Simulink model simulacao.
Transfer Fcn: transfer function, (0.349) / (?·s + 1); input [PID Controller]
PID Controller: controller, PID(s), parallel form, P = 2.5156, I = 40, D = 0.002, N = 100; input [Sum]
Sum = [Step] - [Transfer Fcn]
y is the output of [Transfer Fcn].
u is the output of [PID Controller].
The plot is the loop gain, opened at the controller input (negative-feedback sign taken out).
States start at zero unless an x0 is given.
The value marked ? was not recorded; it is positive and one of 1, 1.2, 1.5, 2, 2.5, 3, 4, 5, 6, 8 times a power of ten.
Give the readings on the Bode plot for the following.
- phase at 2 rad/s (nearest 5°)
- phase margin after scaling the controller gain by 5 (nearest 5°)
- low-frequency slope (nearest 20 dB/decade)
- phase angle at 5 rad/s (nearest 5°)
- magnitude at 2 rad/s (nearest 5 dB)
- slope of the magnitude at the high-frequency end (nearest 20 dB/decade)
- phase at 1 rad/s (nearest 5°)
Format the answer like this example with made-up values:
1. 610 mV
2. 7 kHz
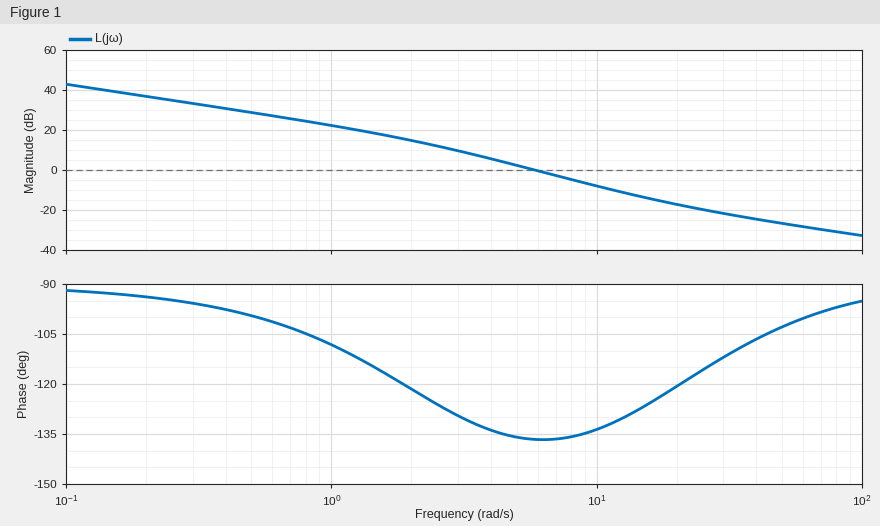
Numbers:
1. -120°
2. 55°
3. -20 dB/decade
4. -135°
5. 15 dB
6. -20 dB/decade
7. -110°
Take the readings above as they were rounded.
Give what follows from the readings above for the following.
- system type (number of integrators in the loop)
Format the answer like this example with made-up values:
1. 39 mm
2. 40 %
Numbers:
1. 1
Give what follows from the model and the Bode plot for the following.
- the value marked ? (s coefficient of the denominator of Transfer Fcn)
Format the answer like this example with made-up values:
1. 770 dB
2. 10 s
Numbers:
1. 0.4
